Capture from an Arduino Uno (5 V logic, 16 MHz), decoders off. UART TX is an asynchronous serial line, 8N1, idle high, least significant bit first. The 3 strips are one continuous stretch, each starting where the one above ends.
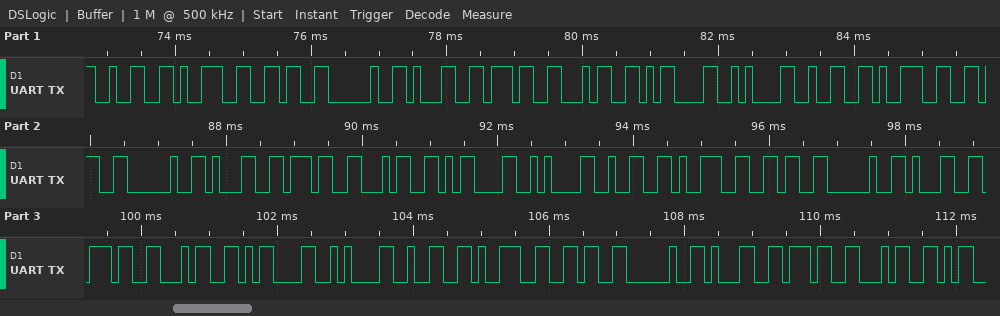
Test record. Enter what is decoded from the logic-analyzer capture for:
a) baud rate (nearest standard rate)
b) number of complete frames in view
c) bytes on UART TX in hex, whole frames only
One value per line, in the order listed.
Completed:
9600 baud
34
32 39 36 20 31 37 34 0D 0A 32 39 36 20 31 37 34 0D 0A 32 39 36 20 31 37 34 0D 0A 32 39 36 20 31 37 34
